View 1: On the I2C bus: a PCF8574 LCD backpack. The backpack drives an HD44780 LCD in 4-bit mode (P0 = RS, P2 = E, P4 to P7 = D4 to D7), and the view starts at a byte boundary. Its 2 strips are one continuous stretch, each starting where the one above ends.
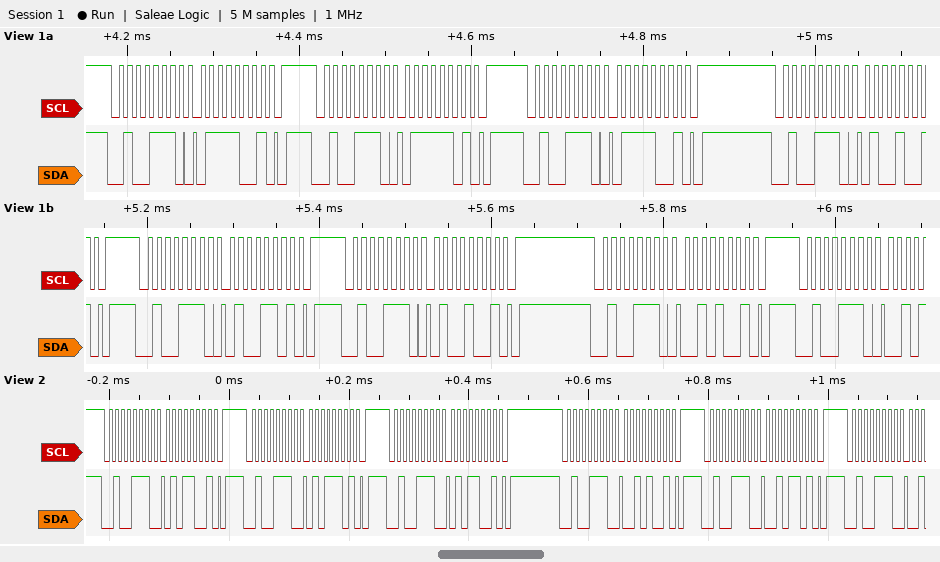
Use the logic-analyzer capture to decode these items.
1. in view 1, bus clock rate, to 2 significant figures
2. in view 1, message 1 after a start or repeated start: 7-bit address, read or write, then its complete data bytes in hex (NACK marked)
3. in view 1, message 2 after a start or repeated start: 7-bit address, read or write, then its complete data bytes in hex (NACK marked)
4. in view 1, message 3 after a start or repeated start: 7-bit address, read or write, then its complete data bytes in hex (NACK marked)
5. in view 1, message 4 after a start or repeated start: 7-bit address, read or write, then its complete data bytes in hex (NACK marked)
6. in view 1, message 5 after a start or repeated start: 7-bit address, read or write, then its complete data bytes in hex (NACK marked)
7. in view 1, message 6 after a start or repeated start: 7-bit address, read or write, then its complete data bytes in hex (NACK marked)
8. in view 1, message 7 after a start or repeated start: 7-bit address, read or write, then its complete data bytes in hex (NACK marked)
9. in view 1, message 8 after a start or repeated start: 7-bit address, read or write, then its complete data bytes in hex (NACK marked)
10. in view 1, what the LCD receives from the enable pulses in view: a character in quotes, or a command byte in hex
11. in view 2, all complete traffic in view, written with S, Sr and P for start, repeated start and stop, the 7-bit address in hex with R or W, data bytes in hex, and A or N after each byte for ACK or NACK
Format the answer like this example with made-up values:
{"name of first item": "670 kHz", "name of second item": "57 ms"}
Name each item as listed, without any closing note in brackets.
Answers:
{"in view 1, bus clock rate, to 2 significant figures": "100 kHz", "in view 1, message 1 after a start or repeated start: 7-bit address, read or write, then its complete data bytes in hex": "0x27 write: 79", "in view 1, message 2 after a start or repeated start: 7-bit address, read or write, then its complete data bytes in hex": "0x27 write: 7D", "in view 1, message 3 after a start or repeated start: 7-bit address, read or write, then its complete data bytes in hex": "0x27 write: 79", "in view 1, message 4 after a start or repeated start: 7-bit address, read or write, then its complete data bytes in hex": "0x27 write: 49", "in view 1, message 5 after a start or repeated start: 7-bit address, read or write, then its complete data bytes in hex": "0x27 write: 4D", "in view 1, message 6 after a start or repeated start: 7-bit address, read or write, then its complete data bytes in hex": "0x27 write: 49", "in view 1, message 7 after a start or repeated start: 7-bit address, read or write, then its complete data bytes in hex": "0x27 write: 29", "in view 1, message 8 after a start or repeated start: 7-bit address, read or write, then its complete data bytes in hex": "0x27 write", "in view 1, what the LCD receives from the enable pulses in view: a character in quotes, or a command byte in hex": "'t'", "in view 2, all complete traffic in view, written with S, Sr and P for start, repeated start and stop, the 7-bit address in hex with R or W, data bytes in hex, and A or N after each byte for ACK or NACK": "S 27W A 59 A P S 27W A 5D A P S 27W A 59 A P S 27W A 29 A P S 27W A 2D A P S 27W A"}
